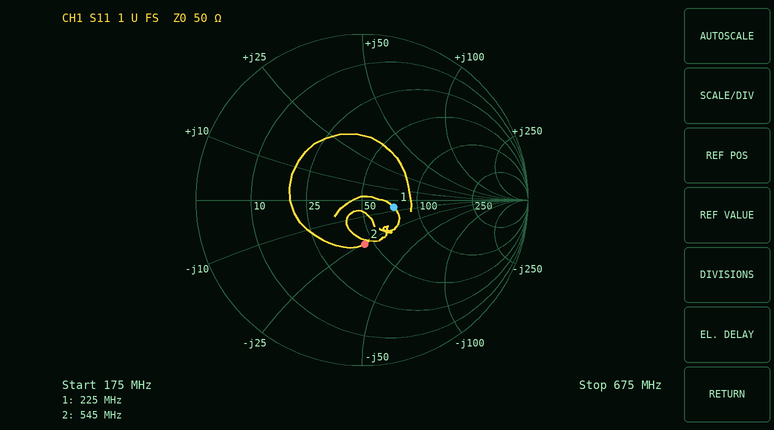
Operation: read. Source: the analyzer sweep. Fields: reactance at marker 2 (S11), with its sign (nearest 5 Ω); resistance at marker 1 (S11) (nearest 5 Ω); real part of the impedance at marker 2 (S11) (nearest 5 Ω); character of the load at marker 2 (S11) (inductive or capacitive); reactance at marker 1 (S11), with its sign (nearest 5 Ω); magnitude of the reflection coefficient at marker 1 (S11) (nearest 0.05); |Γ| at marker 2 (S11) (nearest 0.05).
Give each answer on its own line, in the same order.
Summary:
-25 Ω
75 Ω
45 Ω
capacitive
-5 Ω
0.20
0.25
